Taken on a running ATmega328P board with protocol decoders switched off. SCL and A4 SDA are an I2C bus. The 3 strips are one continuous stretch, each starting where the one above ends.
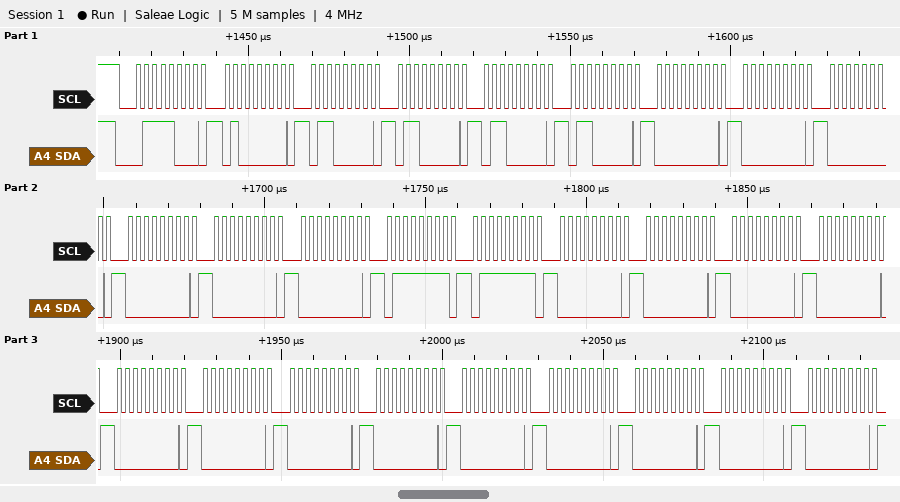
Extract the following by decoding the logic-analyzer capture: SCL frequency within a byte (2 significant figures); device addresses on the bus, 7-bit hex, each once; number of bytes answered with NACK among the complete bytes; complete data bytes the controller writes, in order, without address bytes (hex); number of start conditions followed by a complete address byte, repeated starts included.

400 kHz
0x3C
0
40 60 60 60 60 00 00 00 00 00 00 7F 7F 00 00 00 00 00 00 00 00 00 00 00 00 00
1
